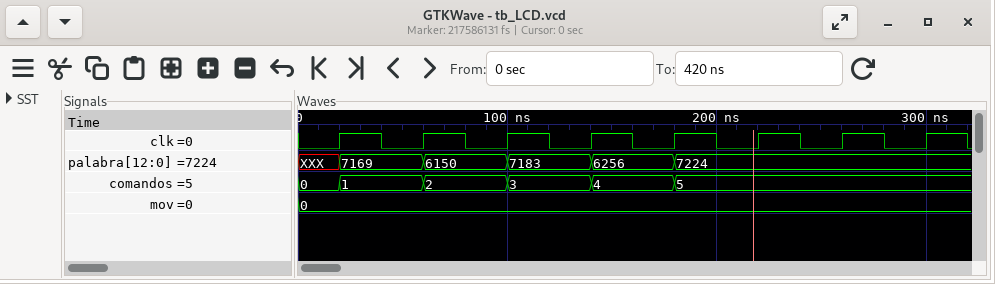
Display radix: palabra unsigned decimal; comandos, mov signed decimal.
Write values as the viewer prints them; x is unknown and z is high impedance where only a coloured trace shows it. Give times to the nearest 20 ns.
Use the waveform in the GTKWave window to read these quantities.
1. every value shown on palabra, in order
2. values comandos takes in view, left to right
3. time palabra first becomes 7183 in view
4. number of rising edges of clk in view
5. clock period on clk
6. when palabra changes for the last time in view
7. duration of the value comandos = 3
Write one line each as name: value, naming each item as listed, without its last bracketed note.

every value shown on palabra, in order: XXX, 7169, 6150, 7183, 6256, 7224
values comandos takes in view, left to right: 0, 1, 2, 3, 4, 5
time palabra first becomes 7183 in view: 100 ns
number of rising edges of clk in view: 8
clock period on clk: 40 ns
when palabra changes for the last time in view: 180 ns
duration of the value comandos = 3: 40 ns
